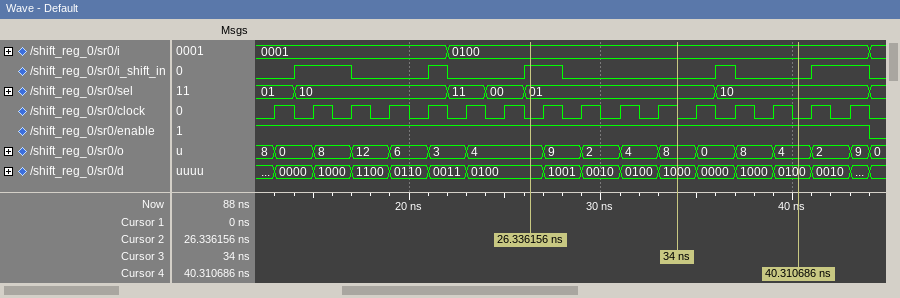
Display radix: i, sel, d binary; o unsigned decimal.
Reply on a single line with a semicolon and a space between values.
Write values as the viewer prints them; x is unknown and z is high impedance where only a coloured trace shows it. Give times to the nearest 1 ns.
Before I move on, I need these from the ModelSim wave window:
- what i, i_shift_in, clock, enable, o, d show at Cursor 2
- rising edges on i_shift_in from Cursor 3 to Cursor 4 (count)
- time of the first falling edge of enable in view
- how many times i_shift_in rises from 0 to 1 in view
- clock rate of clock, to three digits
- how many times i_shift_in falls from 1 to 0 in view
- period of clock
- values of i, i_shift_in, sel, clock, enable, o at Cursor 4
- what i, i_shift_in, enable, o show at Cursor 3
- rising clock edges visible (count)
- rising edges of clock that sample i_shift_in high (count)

i=0100, i_shift_in=1, clock=0, enable=1, o=4, d=0100; 1; 44 ns; 5; 500 MHz; 5; 2 ns; i=0100, i_shift_in=0, sel=10, clock=0, enable=1, o=4; i=0100, i_shift_in=0, enable=1, o=8; 16; 5
